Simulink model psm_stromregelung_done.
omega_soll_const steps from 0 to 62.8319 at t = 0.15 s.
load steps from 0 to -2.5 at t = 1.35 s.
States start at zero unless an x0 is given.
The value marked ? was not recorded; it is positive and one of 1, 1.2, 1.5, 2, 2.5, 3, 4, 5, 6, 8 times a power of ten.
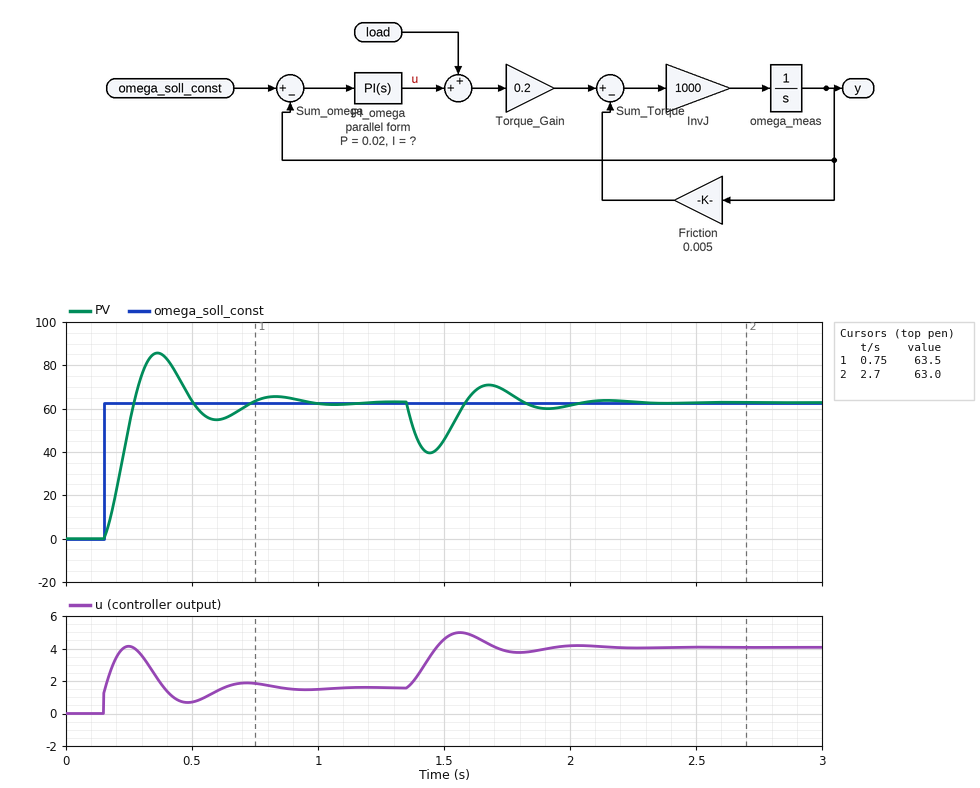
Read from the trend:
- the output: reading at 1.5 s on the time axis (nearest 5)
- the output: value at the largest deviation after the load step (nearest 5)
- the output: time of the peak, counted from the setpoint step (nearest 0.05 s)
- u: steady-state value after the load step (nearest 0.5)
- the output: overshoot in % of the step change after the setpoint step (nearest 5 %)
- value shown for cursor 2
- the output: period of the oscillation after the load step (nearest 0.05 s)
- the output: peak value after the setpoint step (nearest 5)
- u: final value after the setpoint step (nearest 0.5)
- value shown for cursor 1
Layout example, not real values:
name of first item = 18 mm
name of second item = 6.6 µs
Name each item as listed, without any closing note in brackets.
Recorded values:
the output: reading at 1.5 s on the time axis = 45
the output: value at the largest deviation after the load step = 40
the output: time of the peak, counted from the setpoint step = 0.20 s
u: steady-state value after the load step = 4.0
the output: overshoot in % of the step change after the setpoint step = 35 %
value shown for cursor 2 = 63.0
the output: period of the oscillation after the load step = 0.45 s
the output: peak value after the setpoint step = 85
u: final value after the setpoint step = 1.5
value shown for cursor 1 = 63.5
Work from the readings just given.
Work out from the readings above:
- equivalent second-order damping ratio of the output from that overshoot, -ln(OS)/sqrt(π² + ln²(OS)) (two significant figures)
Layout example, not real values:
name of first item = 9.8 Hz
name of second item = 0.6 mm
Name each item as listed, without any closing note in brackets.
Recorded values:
equivalent second-order damping ratio of the output from that overshoot, -ln(OS)/sqrt(π² + ln²(OS)) = 0.32
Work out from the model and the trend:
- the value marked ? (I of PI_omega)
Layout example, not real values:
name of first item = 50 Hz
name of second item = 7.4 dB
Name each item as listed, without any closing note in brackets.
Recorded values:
the value marked ? = 1
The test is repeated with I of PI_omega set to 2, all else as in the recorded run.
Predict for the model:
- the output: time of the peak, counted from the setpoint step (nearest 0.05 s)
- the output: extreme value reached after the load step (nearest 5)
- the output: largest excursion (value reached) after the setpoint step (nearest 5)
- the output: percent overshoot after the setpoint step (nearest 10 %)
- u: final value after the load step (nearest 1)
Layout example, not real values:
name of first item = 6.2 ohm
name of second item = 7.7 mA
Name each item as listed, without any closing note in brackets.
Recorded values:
the output: time of the peak, counted from the setpoint step = 0.15 s
the output: extreme value reached after the load step = 45
the output: largest excursion (value reached) after the setpoint step = 95
the output: percent overshoot after the setpoint step = 50 %
u: final value after the load step = 4
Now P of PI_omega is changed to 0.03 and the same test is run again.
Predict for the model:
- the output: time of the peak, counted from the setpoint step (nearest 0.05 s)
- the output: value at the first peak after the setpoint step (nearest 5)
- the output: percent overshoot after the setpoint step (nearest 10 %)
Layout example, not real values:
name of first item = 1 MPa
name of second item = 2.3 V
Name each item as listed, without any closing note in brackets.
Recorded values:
the output: time of the peak, counted from the setpoint step = 0.20 s
the output: value at the first peak after the setpoint step = 80
the output: percent overshoot after the setpoint step = 30 %
